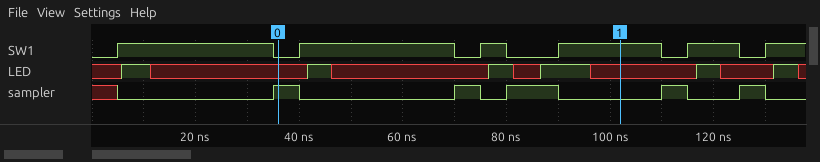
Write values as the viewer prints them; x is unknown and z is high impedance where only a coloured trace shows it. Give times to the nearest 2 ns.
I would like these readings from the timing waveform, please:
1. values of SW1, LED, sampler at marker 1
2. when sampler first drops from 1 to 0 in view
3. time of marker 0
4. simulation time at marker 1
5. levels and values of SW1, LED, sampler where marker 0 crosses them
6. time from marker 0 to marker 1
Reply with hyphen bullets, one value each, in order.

- SW1=1, LED=x, sampler=0
- 40 ns
- 36 ns
- 102 ns
- SW1=0, LED=x, sampler=1
- 66 ns
